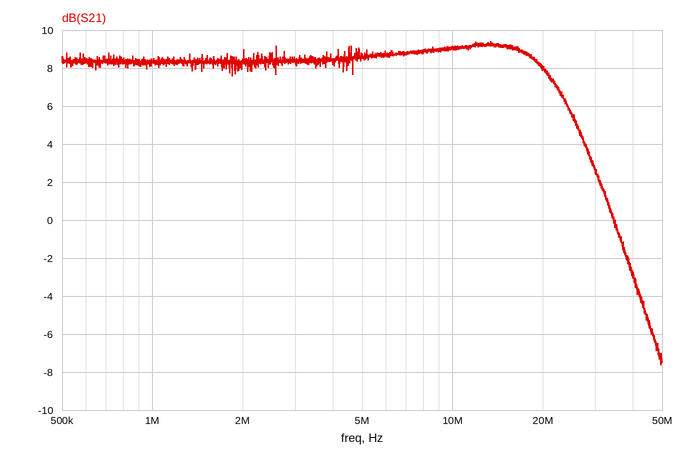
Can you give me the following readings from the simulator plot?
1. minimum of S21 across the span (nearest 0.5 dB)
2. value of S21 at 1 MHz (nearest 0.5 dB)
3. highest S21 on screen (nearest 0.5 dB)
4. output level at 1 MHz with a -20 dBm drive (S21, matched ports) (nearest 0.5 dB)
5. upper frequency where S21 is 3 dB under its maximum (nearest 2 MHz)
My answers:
-7.5 dB
8.5 dB
9.5 dB
-11.5 dBm
24 MHz
